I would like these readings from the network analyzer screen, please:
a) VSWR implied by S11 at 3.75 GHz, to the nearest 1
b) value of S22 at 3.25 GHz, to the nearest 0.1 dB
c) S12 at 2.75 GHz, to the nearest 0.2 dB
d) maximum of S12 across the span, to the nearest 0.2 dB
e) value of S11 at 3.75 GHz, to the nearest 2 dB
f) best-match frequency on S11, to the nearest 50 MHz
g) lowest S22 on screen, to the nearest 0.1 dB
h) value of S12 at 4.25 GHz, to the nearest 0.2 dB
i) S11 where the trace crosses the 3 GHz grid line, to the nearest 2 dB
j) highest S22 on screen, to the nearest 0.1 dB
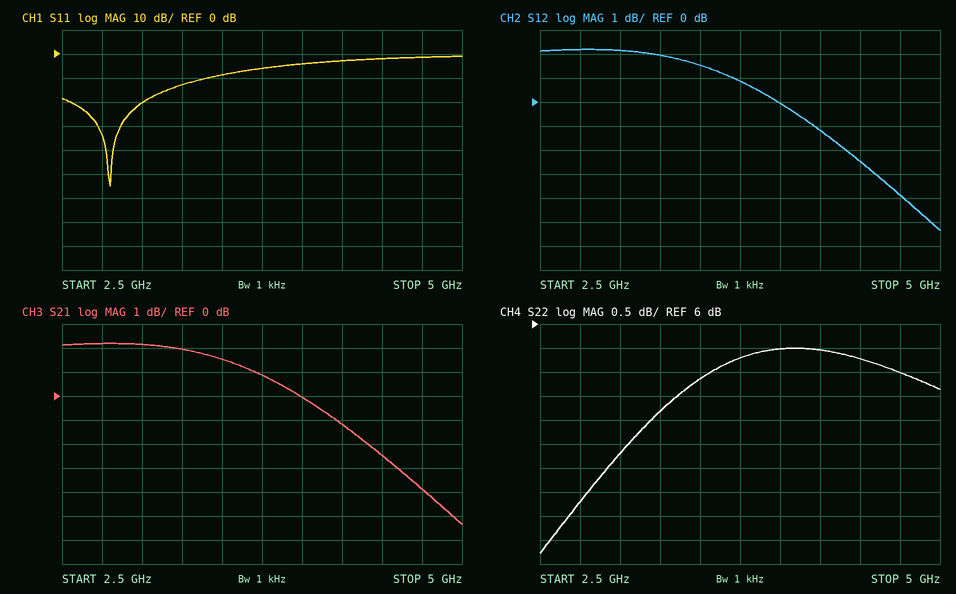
3
4.2 dB
2.2 dB
2.2 dB
-6 dB
2.80 GHz
1.2 dB
-1.2 dB
-20 dB
5.5 dB
